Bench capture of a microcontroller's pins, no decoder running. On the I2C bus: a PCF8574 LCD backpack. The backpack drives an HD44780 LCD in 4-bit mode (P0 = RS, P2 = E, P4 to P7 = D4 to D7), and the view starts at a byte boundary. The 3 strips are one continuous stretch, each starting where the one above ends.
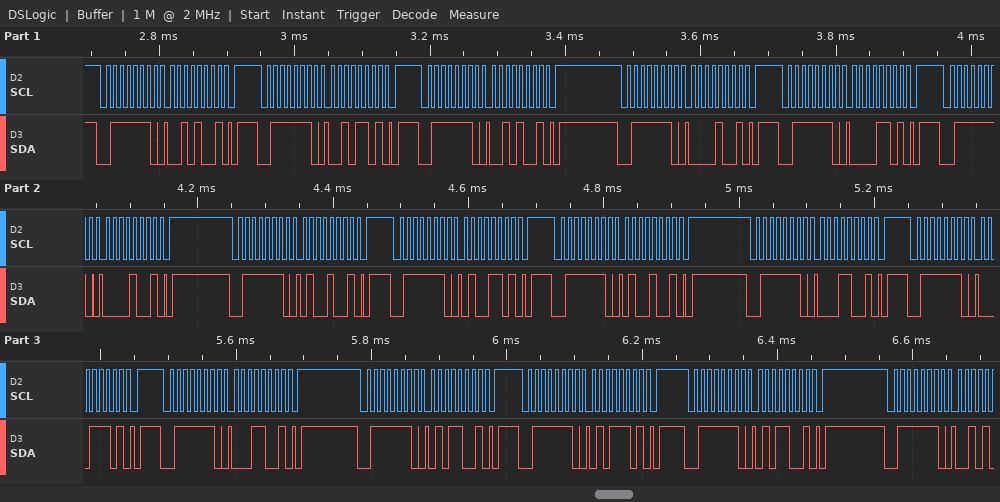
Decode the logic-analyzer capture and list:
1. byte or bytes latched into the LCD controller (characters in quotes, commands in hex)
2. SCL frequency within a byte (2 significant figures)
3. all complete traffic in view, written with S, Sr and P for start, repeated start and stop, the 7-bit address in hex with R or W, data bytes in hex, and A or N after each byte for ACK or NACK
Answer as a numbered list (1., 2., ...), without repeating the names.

1. ' ' 'A'
2. 100 kHz
3. S 3FW A 29 A P S 3FW A 2D A P S 3FW A 29 A P S 3FW A 09 A P S 3FW A 0D A P S 3FW A 09 A P S 3FW A 49 A P S 3FW A 4D A P S 3FW A 49 A P S 3FW A 19 A P S 3FW A 1D A P S 3FW A 19 A P S 3FW A 59 A P S 3FW A 5D A P S 3FW A 59 A P S 3FW A
